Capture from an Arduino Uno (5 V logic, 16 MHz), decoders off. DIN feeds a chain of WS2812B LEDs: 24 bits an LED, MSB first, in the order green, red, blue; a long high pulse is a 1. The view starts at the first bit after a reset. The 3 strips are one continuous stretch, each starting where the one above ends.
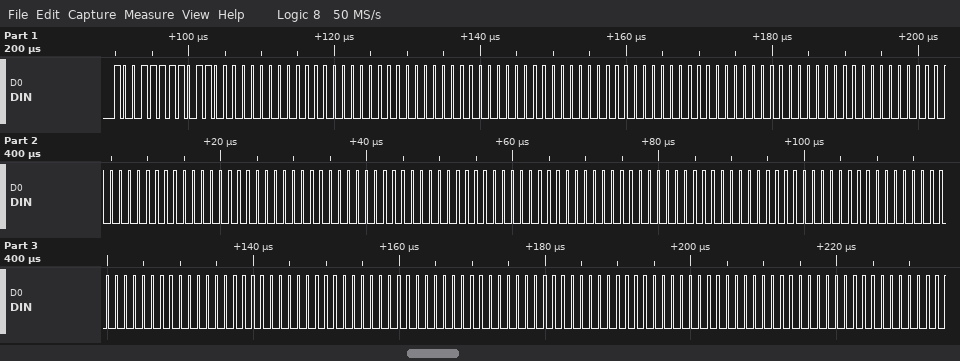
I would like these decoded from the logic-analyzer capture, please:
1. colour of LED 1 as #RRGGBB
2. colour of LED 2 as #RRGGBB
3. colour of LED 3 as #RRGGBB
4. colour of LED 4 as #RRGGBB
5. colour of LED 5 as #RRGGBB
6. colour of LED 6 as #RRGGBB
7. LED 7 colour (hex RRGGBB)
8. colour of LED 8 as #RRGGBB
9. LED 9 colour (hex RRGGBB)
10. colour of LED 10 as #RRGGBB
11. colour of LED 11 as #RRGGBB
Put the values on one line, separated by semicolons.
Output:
#609F00; #000000; #000000; #000000; #000000; #000000; #000000; #000000; #000000; #000000; #000000
